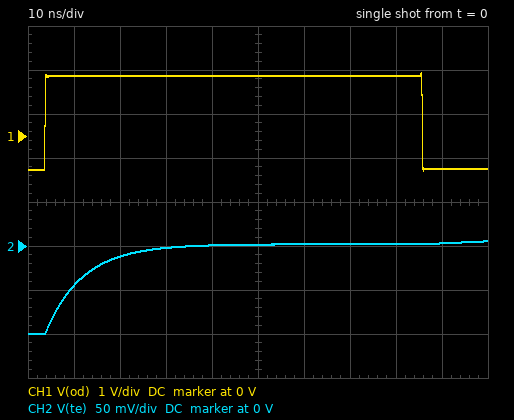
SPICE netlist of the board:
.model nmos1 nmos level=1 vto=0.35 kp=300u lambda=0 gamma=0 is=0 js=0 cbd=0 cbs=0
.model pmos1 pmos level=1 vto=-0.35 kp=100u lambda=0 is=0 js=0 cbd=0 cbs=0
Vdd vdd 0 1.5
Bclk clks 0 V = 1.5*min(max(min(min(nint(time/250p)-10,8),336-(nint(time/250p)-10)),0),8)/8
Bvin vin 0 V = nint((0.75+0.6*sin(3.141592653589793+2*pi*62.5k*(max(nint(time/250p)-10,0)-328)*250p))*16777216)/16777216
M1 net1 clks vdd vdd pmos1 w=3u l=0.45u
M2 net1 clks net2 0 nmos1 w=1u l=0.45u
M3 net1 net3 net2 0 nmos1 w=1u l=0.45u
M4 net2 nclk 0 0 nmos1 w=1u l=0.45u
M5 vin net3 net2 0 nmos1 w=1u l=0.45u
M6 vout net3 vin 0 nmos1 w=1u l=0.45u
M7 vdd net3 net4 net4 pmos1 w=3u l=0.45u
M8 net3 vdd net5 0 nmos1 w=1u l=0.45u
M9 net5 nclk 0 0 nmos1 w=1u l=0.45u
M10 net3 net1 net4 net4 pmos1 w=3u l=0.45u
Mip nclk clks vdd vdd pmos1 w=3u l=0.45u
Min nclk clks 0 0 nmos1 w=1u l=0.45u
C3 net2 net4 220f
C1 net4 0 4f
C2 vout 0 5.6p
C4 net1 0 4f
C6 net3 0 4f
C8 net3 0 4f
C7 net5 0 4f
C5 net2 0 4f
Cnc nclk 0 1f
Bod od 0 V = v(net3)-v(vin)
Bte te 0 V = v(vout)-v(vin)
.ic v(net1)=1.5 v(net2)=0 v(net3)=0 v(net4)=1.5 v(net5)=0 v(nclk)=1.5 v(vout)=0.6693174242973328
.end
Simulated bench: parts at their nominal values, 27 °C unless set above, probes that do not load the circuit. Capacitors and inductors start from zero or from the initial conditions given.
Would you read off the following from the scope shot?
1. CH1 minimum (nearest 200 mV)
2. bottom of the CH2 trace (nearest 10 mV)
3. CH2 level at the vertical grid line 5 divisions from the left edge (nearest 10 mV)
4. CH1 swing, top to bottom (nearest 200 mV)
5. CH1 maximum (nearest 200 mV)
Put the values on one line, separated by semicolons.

-800 mV; -100 mV; 0 V; 2.2 V; 1.4 V
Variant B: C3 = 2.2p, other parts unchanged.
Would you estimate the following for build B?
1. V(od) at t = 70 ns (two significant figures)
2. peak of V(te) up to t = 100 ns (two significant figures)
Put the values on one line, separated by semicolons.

1.5 V; 5.1 mV
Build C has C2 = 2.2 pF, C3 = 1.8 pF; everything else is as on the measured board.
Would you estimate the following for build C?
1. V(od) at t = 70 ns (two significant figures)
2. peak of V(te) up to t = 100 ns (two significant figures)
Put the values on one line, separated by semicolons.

1.5 V; 4.1 mV
